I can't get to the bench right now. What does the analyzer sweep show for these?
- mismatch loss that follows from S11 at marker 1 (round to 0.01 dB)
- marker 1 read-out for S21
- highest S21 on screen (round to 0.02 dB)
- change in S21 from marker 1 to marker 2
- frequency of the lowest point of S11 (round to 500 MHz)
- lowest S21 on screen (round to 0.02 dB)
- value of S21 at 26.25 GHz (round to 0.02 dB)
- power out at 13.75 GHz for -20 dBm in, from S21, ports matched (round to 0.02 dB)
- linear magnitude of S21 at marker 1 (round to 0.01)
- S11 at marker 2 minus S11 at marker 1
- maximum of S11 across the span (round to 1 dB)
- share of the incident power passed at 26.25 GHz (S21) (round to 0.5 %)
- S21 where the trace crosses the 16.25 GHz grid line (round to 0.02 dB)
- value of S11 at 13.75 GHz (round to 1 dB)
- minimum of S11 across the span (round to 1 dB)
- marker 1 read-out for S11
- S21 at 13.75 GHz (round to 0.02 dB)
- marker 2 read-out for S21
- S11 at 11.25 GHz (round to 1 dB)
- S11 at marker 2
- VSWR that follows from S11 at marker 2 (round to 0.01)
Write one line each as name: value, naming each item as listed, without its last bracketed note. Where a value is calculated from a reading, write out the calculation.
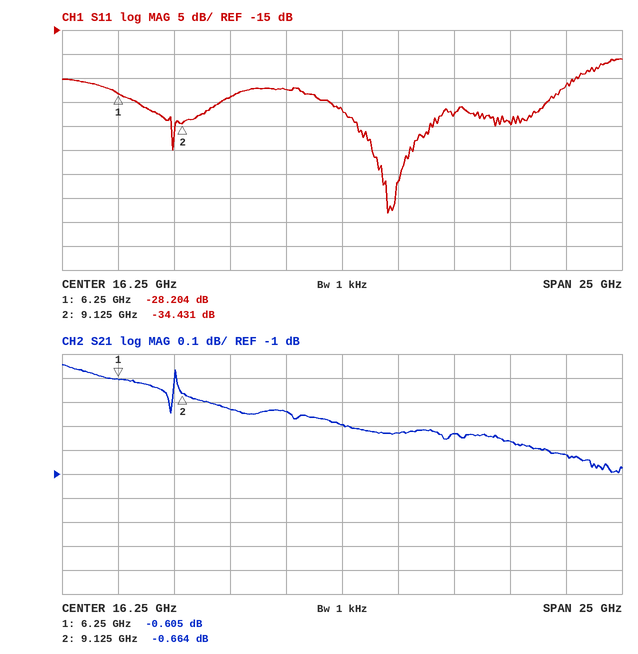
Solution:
mismatch loss that follows from S11 at marker 1: −10 log10(1 − 10^(-28.204/10)) ≈ 0.01 dB
marker 1 read-out for S21: -0.605 dB
highest S21 on screen: -0.54 dB
change in S21 from marker 1 to marker 2: -0.664 − (-0.605) = -0.059 dB
frequency of the lowest point of S11: 18.5 GHz
lowest S21 on screen: -1.00 dB
value of S21 at 26.25 GHz: -0.92 dB
power out at 13.75 GHz for -20 dBm in, from S21, ports matched: -20 dBm + (-0.74 dB) = -20.74 dBm
linear magnitude of S21 at marker 1: 10^(-0.605/20) ≈ 0.93
S11 at marker 2 minus S11 at marker 1: -34.431 − (-28.204) = -6.227 dB
maximum of S11 across the span: -21 dB
share of the incident power passed at 26.25 GHz (S21): 10^(-0.92/10) ≈ 80.9 %, so 81.0 % to the nearest 0.5 %
S21 where the trace crosses the 16.25 GHz grid line: -0.80 dB
value of S11 at 13.75 GHz: -27 dB
minimum of S11 across the span: -53 dB
marker 1 read-out for S11: -28.204 dB
S21 at 13.75 GHz: -0.74 dB
marker 2 read-out for S21: -0.664 dB
S11 at 11.25 GHz: -29 dB
S11 at marker 2: -34.431 dB
VSWR that follows from S11 at marker 2: (1 + 0.0190)/(1 − 0.0190) ≈ 1.04
